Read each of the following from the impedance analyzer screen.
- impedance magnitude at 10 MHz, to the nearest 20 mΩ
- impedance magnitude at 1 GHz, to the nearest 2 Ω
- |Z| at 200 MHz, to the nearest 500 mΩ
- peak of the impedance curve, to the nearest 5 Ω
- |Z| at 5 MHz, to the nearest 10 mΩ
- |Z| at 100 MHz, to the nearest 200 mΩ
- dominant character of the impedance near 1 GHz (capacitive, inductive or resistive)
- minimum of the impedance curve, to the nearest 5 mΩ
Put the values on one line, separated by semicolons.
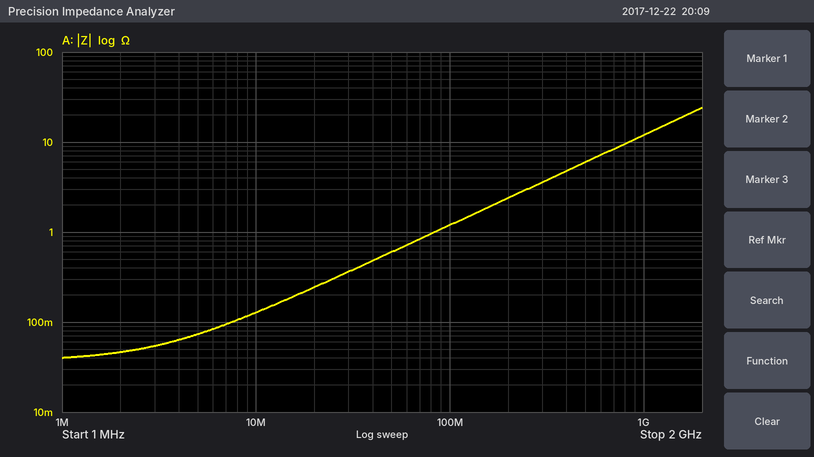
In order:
120 mΩ; 12 Ω; 2.5 Ω; 25 Ω; 70 mΩ; 1.2 Ω; inductive; 40 mΩ
